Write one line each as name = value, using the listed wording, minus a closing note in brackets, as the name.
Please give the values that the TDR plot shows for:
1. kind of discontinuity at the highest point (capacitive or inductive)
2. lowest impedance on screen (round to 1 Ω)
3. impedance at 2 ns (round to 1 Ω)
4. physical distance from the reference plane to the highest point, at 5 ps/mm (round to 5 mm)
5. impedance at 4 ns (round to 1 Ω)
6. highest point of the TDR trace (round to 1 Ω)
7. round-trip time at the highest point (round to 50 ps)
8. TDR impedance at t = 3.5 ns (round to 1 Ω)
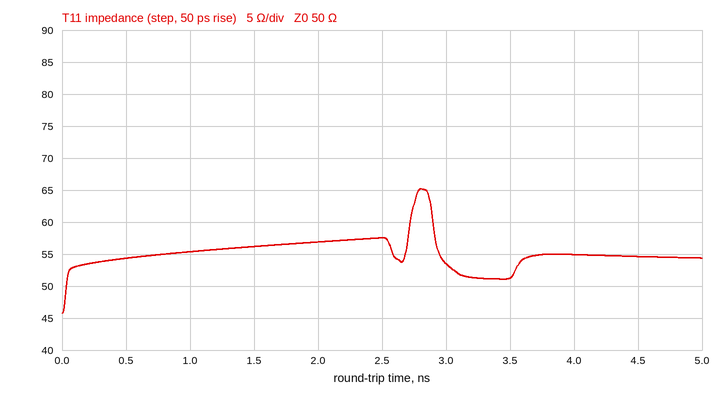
kind of discontinuity at the highest point = inductive
lowest impedance on screen = 46 Ω
impedance at 2 ns = 57 Ω
physical distance from the reference plane to the highest point, at 5 ps/mm = 280 mm
impedance at 4 ns = 55 Ω
highest point of the TDR trace = 65 Ω
round-trip time at the highest point = 2.80 ns
TDR impedance at t = 3.5 ns = 51 Ω
